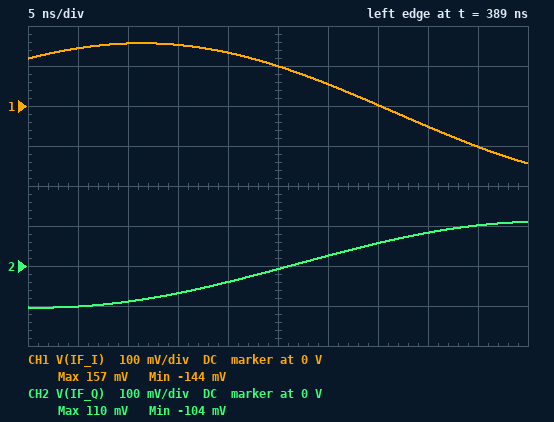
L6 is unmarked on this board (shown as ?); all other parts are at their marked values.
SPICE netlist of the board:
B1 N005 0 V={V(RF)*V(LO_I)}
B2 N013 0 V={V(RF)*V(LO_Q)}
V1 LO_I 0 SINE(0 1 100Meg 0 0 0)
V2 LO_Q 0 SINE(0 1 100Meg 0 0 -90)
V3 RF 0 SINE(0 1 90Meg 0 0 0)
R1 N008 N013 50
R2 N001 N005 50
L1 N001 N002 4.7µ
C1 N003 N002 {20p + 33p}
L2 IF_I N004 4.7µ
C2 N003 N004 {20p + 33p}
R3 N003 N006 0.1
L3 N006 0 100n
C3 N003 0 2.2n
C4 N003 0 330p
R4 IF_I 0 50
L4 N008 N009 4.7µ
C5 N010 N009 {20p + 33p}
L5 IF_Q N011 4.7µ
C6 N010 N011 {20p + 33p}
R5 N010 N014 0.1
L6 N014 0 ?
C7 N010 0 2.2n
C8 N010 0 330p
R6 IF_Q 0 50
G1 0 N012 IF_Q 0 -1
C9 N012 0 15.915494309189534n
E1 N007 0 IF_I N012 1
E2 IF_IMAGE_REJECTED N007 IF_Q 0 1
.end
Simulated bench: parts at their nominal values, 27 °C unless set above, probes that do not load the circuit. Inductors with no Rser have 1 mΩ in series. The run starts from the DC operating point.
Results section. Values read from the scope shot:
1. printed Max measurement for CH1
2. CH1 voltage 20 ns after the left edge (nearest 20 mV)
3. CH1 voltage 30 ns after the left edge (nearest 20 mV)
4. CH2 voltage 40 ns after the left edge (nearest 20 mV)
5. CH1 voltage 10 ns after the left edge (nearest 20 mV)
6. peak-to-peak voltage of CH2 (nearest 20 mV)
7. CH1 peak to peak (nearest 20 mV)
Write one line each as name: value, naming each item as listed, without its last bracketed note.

printed Max measurement for CH1: 157 mV
CH1 voltage 20 ns after the left edge: 140 mV
CH1 voltage 30 ns after the left edge: 60 mV
CH2 voltage 40 ns after the left edge: 80 mV
CH1 voltage 10 ns after the left edge: 160 mV
peak-to-peak voltage of CH2: 220 mV
CH1 peak to peak: 300 mV
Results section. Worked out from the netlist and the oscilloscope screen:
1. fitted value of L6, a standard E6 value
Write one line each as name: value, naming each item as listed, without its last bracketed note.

fitted value of L6, a standard E6 value: 150 nH
